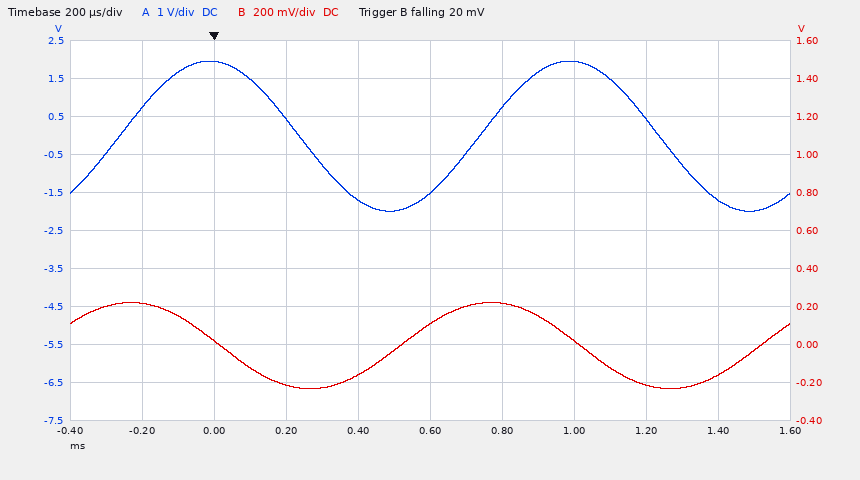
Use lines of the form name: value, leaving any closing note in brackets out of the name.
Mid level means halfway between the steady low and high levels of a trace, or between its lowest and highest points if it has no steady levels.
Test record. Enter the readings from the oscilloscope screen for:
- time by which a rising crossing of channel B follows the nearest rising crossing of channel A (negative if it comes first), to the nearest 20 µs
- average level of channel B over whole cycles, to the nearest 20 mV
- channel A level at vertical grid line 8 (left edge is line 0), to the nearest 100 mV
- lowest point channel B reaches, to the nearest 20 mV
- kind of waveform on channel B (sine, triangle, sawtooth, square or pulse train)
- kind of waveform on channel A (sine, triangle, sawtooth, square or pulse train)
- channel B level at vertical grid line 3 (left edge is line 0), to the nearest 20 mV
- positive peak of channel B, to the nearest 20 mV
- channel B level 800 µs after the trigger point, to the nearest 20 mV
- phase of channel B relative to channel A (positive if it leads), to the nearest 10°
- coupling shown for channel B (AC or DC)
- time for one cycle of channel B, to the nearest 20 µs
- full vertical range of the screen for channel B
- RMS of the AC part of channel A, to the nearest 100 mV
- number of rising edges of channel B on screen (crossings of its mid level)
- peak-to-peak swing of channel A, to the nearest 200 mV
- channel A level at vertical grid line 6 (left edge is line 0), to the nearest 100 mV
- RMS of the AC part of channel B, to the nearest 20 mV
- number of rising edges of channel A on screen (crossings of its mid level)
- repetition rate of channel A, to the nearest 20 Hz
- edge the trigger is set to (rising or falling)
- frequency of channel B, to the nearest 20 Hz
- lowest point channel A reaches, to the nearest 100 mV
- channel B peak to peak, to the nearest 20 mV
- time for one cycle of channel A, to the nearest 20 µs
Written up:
time by which a rising crossing of channel B follows the nearest rising crossing of channel A (negative if it comes first), to the nearest 20 µs: -220 µs
average level of channel B over whole cycles, to the nearest 20 mV: 0 mV
channel A level at vertical grid line 8 (left edge is line 0), to the nearest 100 mV: 400 mV
lowest point channel B reaches, to the nearest 20 mV: -240 mV
kind of waveform on channel B: sine
kind of waveform on channel A: sine
channel B level at vertical grid line 3 (left edge is line 0), to the nearest 20 mV: -220 mV
positive peak of channel B, to the nearest 20 mV: 220 mV
channel B level 800 µs after the trigger point, to the nearest 20 mV: 220 mV
phase of channel B relative to channel A (positive if it leads), to the nearest 10°: +80°
coupling shown for channel B: DC
time for one cycle of channel B, to the nearest 20 µs: 1.00 ms
full vertical range of the screen for channel B: 2 V
RMS of the AC part of channel A, to the nearest 100 mV: 1.4 V
number of rising edges of channel B on screen: 2
peak-to-peak swing of channel A, to the nearest 200 mV: 4.0 V
channel A level at vertical grid line 6 (left edge is line 0), to the nearest 100 mV: 700 mV
RMS of the AC part of channel B, to the nearest 20 mV: 160 mV
number of rising edges of channel A on screen: 2
repetition rate of channel A, to the nearest 20 Hz: 1.00 kHz
edge the trigger is set to: falling
frequency of channel B, to the nearest 20 Hz: 1.00 kHz
lowest point channel A reaches, to the nearest 100 mV: -2.0 V
channel B peak to peak, to the nearest 20 mV: 460 mV
time for one cycle of channel A, to the nearest 20 µs: 1.00 ms
